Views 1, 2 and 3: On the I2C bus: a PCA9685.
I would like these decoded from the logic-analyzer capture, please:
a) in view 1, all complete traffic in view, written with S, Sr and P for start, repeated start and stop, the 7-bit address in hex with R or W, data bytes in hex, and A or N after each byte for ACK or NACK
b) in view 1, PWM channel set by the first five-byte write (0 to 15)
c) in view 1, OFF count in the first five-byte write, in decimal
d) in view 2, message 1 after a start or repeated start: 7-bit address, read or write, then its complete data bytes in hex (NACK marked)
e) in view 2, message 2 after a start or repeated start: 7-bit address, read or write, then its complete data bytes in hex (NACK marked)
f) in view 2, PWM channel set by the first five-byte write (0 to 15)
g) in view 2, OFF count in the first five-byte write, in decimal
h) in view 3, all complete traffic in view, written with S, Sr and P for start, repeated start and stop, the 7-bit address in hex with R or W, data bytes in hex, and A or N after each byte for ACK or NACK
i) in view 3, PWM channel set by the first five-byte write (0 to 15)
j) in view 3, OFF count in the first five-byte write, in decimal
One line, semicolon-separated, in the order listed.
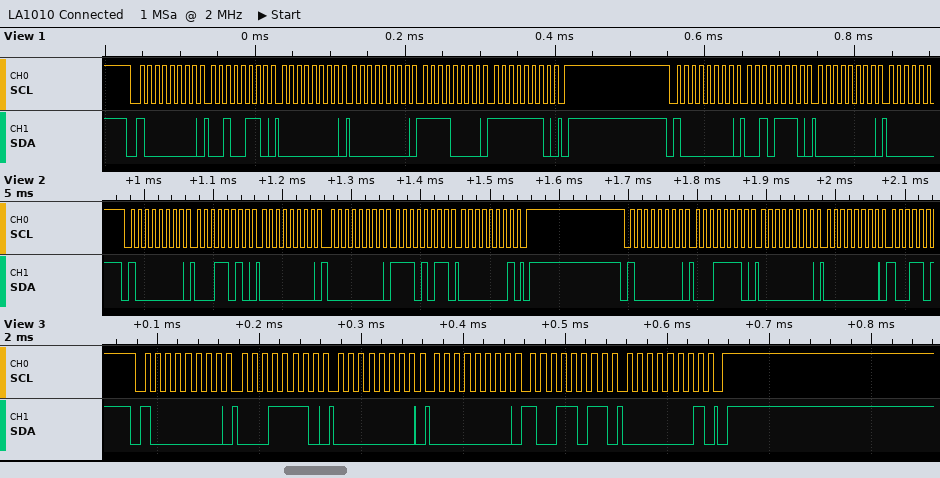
S 40W A 26 A 00 A 00 A F0 A FE A P S 40W A 2E A 00 A; 8; 65264; 0x40 write: 1A 00 00 EB 01; 0x40 write: 1E 00 00; 5; 491; S 40W A 1E A 00 A 00 A 9B A 01 A P; 6; 411
